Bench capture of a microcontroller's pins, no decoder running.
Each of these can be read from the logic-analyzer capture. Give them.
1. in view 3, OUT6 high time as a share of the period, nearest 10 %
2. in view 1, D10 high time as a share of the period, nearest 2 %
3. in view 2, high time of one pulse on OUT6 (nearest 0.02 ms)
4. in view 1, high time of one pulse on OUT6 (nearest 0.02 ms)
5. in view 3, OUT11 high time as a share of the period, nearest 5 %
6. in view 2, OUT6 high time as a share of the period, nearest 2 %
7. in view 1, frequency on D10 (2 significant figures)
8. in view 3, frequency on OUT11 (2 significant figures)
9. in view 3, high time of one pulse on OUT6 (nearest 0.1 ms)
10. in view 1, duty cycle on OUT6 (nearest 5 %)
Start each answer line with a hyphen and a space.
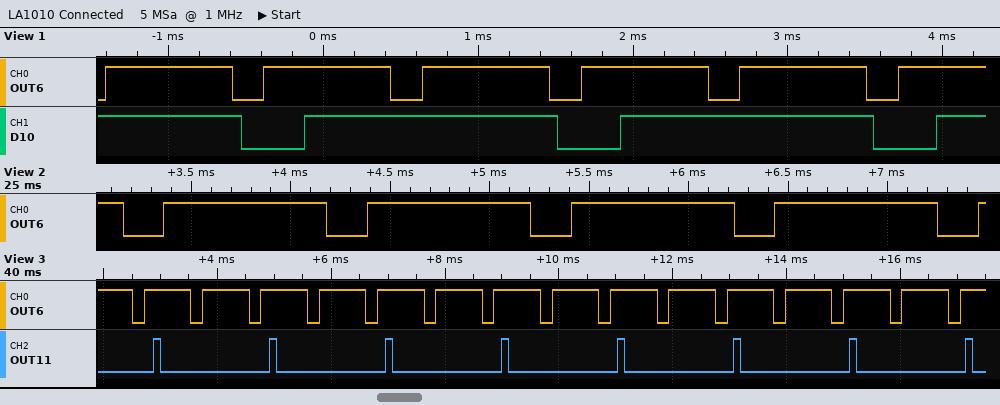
- 80 %
- 80 %
- 0.82 ms
- 0.82 ms
- 5 %
- 80 %
- 490 Hz
- 490 Hz
- 0.8 ms
- 80 %
